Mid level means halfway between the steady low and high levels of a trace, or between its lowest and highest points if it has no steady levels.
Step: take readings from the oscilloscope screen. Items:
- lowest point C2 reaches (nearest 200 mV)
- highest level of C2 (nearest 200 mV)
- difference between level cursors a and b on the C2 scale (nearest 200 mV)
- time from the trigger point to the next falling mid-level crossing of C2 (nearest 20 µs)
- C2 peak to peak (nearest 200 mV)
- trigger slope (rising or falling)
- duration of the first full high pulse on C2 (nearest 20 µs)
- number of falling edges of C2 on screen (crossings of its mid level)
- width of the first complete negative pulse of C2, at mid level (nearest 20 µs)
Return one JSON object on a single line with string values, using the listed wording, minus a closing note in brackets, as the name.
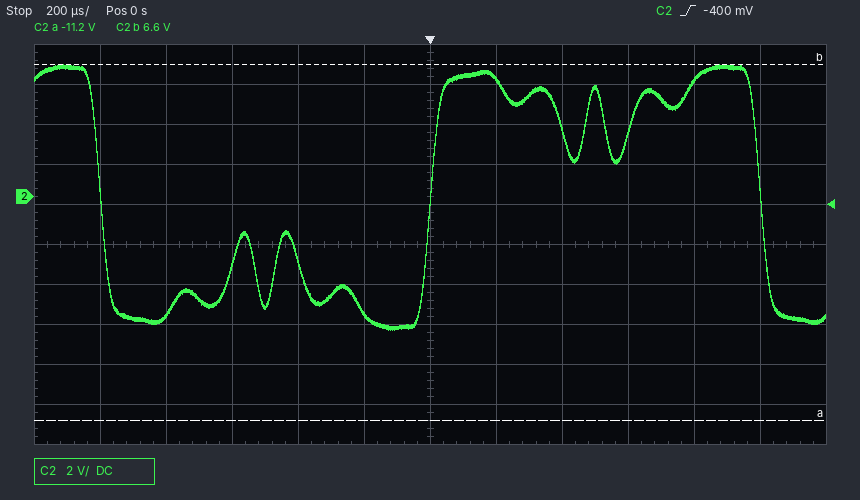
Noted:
{"lowest point C2 reaches": "-6.6 V", "highest level of C2": "6.6 V", "difference between level cursors a and b on the C2 scale": "17.8 V", "time from the trigger point to the next falling mid-level crossing of C2": "1.00 ms", "C2 peak to peak": "13.2 V", "trigger slope": "rising", "duration of the first full high pulse on C2": "1.00 ms", "number of falling edges of C2 on screen": "2", "width of the first complete negative pulse of C2, at mid level": "1.00 ms"}
